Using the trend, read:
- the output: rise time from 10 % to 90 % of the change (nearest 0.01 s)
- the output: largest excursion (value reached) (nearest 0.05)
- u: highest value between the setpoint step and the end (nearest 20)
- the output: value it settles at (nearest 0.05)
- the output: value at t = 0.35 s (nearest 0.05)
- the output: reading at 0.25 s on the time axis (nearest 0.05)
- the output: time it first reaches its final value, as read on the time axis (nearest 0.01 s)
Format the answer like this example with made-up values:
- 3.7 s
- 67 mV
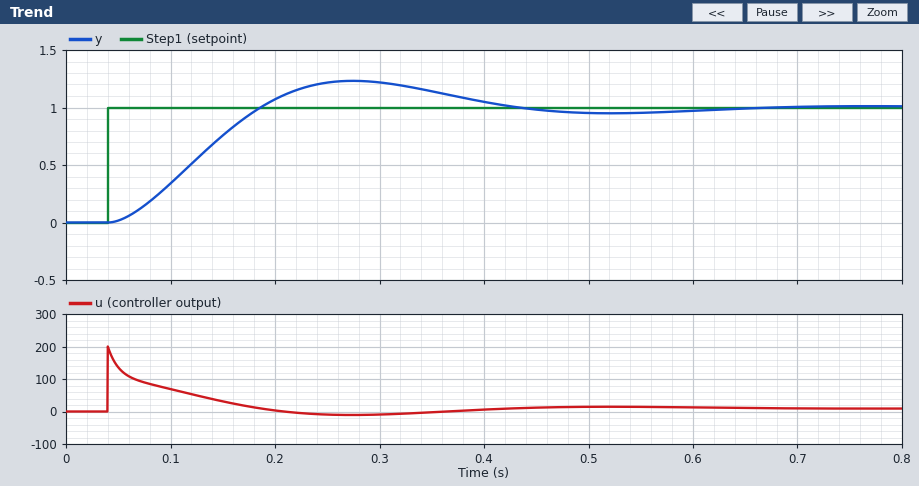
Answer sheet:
- 0.10 s
- 1.25
- 200
- 1.00
- 1.15
- 1.20
- 0.19 s
